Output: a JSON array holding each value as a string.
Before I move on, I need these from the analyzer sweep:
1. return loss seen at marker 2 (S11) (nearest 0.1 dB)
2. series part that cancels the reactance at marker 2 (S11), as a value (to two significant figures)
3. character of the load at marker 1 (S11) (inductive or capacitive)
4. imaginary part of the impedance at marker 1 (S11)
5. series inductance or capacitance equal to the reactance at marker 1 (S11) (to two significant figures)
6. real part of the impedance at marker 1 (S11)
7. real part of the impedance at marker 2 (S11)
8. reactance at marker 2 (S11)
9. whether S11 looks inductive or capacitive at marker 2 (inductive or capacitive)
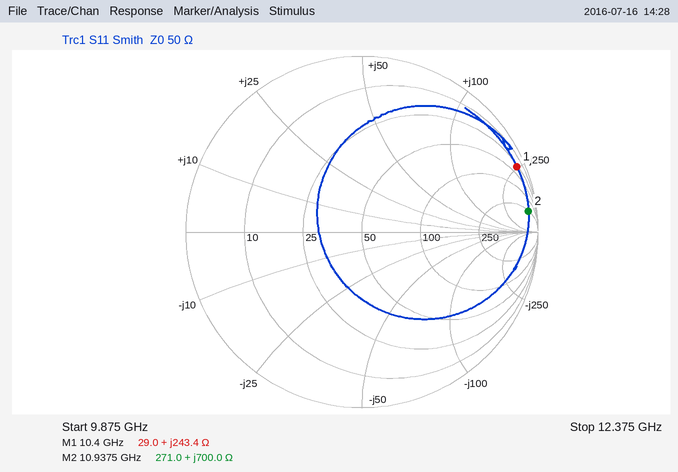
["0.4 dB", "21 fF", "inductive", "+243.4 Ω", "3.7 nH", "29.0 Ω", "271.0 Ω", "+700.0 Ω", "inductive"]
